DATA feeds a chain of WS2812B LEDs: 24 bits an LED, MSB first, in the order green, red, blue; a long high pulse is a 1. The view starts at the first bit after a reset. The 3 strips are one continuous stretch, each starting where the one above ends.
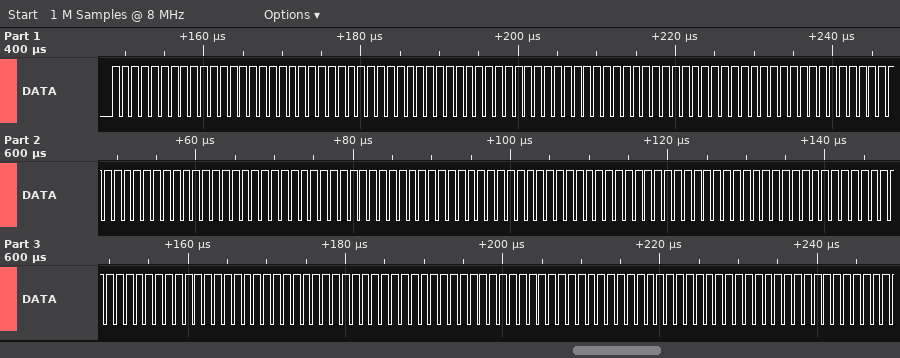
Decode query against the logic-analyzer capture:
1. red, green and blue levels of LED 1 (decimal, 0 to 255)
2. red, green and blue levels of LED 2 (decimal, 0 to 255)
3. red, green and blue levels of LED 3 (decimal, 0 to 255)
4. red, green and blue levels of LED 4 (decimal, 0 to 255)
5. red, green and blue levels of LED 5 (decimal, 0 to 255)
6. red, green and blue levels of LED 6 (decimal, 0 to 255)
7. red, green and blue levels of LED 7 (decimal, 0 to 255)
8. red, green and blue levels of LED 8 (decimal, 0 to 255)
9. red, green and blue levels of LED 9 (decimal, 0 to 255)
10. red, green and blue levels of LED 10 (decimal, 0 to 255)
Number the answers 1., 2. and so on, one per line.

1. 255, 255, 255
2. 255, 255, 255
3. 255, 255, 255
4. 255, 255, 255
5. 255, 255, 255
6. 255, 255, 255
7. 255, 255, 255
8. 255, 255, 255
9. 255, 255, 255
10. 255, 255, 255
